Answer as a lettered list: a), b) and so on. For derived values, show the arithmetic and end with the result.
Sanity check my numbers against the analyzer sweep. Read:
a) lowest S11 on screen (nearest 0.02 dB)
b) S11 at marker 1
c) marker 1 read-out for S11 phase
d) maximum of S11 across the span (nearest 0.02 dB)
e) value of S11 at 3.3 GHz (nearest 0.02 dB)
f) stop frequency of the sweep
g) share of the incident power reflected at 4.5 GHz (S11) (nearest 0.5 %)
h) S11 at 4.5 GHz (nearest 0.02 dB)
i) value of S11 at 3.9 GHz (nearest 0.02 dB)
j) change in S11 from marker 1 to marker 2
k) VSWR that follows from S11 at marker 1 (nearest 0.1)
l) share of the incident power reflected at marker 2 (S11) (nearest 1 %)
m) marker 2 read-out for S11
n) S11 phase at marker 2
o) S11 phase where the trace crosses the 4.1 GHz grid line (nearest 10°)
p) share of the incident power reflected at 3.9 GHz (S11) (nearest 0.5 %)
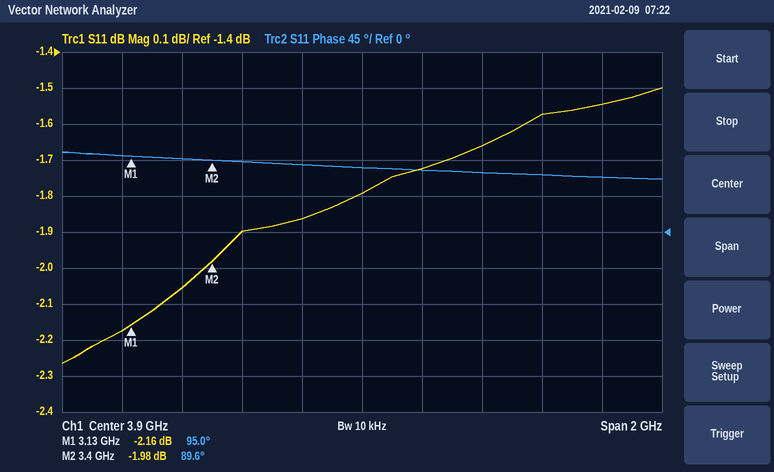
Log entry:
a) -2.26 dB
b) -2.16 dB
c) 95.0°
d) -1.50 dB
e) -2.06 dB
f) 4.9 GHz
g) 10^(-1.58/10) ≈ 69.5 %
h) -1.58 dB
i) -1.80 dB
j) -1.98 − (-2.16) = 0.18 dB
k) (1 + 0.7798)/(1 − 0.7798) ≈ 8.1
l) 10^(-1.98/10) ≈ 63 %
m) -1.98 dB
n) 89.6°
o) 80°
p) 10^(-1.8/10) ≈ 66.1 %, so 66.0 % to the nearest 0.5 %
